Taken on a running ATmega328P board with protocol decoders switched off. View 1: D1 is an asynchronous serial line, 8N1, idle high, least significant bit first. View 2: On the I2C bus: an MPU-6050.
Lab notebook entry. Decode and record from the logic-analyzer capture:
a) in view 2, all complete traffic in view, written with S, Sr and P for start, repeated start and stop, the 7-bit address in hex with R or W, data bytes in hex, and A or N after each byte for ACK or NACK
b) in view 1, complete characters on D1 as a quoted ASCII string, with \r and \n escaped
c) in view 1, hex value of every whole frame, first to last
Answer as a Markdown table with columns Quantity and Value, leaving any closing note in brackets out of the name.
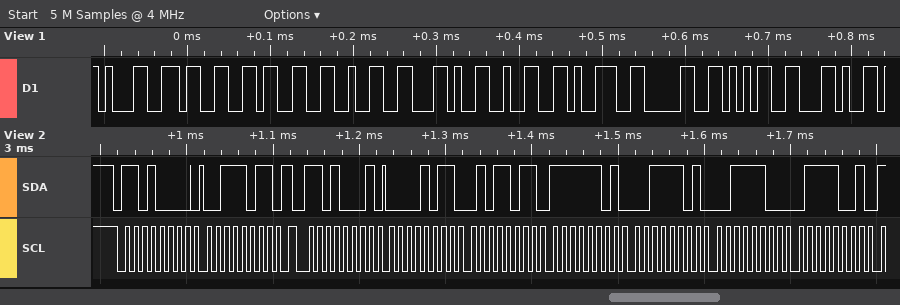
| Quantity | Value |
|---|---|
| in view 2, all complete traffic in view, written with S, Sr and P for start, repeated start and stop, the 7-bit address in hex with R or W, data bytes in hex, and A or N after each byte for ACK or NACK | S 68W A 3B A Sr 68R A 0B A 5B A FD A 3D A 3C A 79 A |
| in view 1, complete characters on D1 as a quoted ASCII string, with \r and \n escaped | "1332,2905," |
| in view 1, hex value of every whole frame, first to last | 31 33 33 32 2C 32 39 30 35 2C |
